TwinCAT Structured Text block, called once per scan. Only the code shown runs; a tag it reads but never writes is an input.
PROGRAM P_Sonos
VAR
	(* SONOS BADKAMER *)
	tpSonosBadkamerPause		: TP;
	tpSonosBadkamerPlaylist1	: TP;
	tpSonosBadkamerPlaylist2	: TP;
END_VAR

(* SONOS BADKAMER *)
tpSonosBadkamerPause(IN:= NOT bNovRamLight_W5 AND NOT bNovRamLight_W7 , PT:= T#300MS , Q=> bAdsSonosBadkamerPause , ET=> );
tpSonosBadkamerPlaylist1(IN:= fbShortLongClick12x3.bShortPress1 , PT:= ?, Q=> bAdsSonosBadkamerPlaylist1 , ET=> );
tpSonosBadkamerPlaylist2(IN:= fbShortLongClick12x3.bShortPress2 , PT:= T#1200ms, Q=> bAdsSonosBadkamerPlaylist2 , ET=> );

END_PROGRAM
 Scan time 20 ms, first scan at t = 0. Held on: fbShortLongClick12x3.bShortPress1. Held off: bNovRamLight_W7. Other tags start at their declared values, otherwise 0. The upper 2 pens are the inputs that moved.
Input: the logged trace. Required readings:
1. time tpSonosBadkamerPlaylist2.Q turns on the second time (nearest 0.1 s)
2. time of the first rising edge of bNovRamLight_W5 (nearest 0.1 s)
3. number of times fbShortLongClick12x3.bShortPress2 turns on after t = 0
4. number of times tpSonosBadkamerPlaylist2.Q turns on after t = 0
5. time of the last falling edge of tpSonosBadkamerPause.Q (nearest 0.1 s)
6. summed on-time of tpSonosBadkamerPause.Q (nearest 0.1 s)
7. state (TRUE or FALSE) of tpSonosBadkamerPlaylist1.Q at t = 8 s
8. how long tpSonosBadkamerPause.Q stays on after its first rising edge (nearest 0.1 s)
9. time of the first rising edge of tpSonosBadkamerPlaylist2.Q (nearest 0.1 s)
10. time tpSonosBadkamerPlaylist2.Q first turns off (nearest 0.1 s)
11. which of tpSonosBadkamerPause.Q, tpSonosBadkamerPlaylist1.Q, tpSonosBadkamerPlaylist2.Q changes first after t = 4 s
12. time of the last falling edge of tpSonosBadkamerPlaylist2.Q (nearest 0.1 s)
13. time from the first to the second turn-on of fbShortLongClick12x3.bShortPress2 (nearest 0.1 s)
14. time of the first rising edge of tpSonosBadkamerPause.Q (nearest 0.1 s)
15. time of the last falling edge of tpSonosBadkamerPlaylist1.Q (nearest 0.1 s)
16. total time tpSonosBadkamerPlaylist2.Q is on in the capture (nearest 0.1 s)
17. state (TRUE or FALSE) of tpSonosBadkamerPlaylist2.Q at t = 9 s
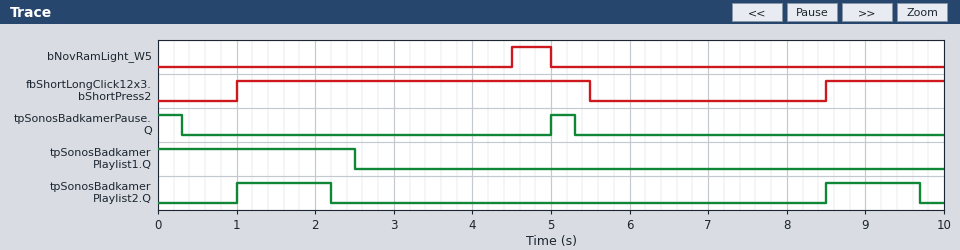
8.5 s
4.5 s
2
2
5.3 s
0.6 s
FALSE
0.3 s
1.0 s
2.2 s
tpSonosBadkamerPause.Q
9.7 s
7.5 s
5.0 s
2.5 s
2.4 s
TRUE
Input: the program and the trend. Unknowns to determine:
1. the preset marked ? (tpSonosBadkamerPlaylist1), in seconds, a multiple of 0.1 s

2.5 s
